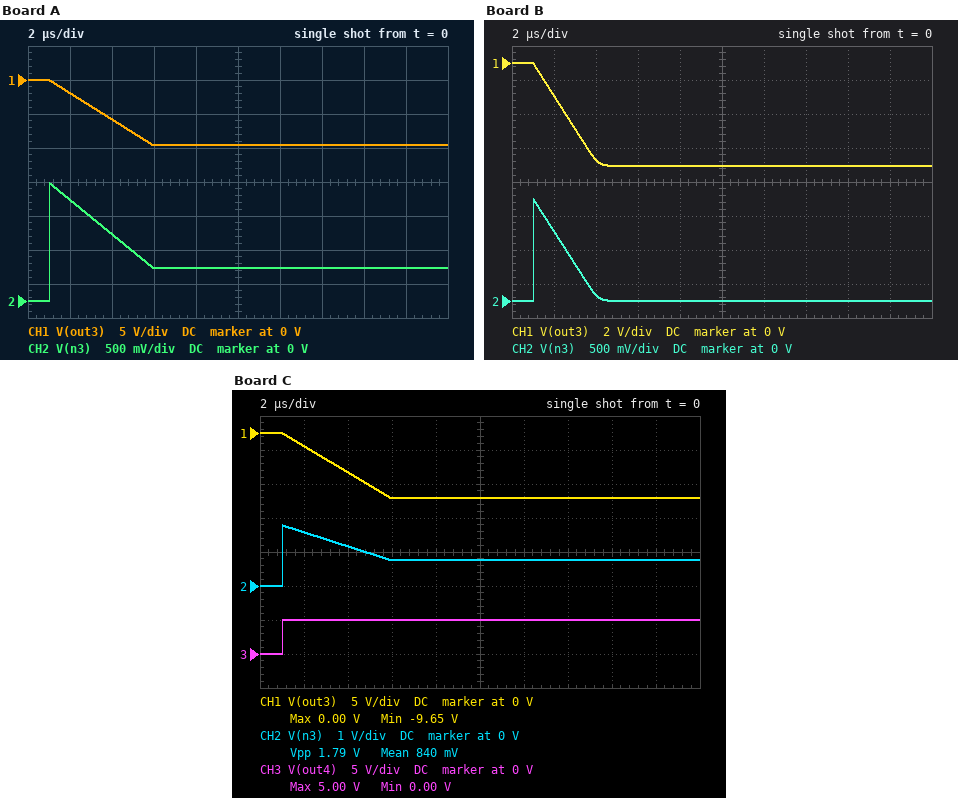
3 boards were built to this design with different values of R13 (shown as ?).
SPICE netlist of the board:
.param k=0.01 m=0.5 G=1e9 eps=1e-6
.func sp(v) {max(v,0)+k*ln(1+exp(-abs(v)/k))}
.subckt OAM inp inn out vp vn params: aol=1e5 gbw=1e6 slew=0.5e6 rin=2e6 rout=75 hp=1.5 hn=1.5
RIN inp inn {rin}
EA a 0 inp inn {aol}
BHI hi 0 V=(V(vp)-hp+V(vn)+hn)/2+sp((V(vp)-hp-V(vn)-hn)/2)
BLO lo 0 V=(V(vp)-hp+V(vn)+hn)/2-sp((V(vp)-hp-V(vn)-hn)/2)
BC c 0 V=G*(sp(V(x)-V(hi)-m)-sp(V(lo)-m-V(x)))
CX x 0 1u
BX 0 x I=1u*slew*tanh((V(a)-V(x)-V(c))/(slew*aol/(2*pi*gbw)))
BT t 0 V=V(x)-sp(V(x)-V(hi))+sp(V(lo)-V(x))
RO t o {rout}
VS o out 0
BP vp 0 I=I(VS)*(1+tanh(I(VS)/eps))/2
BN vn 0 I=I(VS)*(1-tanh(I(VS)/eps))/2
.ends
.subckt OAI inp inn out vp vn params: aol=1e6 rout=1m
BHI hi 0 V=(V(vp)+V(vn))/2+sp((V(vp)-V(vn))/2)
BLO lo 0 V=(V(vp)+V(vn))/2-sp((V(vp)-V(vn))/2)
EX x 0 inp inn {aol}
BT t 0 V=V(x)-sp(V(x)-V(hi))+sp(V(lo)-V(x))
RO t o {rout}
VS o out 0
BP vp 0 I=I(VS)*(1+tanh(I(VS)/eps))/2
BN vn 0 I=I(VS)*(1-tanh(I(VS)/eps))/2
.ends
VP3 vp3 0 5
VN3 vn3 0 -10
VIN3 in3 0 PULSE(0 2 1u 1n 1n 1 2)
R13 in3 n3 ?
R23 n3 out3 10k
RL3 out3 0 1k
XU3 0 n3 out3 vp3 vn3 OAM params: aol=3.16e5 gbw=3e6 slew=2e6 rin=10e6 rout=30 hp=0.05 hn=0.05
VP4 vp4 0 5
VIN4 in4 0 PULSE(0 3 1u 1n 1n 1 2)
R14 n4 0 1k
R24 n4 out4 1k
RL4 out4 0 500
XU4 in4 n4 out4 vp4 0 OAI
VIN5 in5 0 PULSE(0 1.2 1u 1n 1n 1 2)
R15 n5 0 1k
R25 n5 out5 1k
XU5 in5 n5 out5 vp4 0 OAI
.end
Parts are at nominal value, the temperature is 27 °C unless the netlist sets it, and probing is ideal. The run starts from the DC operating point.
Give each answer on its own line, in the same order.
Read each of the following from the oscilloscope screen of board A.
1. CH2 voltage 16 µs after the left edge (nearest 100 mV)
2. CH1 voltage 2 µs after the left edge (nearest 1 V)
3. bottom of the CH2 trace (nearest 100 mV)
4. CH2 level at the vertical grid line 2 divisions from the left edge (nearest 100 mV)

500 mV
-2 V
0 V
1.0 V
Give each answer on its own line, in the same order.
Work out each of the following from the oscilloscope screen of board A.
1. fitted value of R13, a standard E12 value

1.5 kΩ
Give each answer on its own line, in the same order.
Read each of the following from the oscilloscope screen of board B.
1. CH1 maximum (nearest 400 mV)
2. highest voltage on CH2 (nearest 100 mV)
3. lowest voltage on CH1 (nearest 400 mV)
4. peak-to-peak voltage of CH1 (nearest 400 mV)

0 V
1.5 V
-6.0 V
6.0 V
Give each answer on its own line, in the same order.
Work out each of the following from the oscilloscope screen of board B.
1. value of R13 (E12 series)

3.3 kΩ
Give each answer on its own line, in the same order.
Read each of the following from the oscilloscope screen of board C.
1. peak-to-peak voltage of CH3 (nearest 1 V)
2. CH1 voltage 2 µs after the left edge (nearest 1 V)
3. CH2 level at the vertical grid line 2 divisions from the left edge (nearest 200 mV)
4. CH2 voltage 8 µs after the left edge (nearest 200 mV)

5 V
-2 V
1.2 V
800 mV
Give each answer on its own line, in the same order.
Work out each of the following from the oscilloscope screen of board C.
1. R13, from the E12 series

1.2 kΩ
